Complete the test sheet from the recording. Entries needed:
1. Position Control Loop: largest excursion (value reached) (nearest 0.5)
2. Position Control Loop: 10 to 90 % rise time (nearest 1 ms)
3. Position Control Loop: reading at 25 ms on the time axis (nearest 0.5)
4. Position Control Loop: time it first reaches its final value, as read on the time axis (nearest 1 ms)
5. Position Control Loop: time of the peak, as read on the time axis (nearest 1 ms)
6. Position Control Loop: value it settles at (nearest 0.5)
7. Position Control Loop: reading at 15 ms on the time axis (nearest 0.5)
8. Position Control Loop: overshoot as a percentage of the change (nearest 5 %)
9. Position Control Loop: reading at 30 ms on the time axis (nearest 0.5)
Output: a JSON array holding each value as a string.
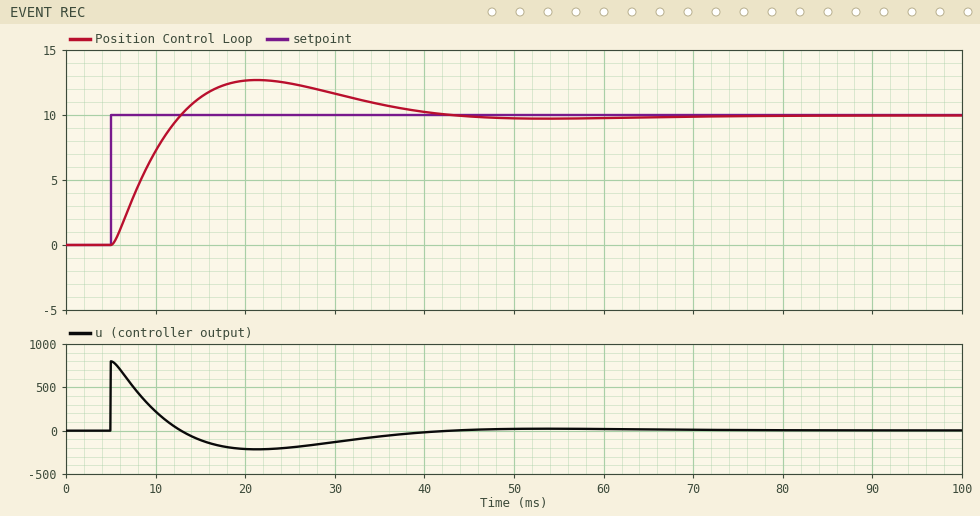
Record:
["12.5", "6 ms", "12.5", "13 ms", "21 ms", "10.0", "11.5", "25 %", "11.5"]
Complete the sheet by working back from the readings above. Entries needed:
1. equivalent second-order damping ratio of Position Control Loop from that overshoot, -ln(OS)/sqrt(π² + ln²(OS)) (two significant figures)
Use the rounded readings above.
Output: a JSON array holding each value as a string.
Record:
["0.40"]
